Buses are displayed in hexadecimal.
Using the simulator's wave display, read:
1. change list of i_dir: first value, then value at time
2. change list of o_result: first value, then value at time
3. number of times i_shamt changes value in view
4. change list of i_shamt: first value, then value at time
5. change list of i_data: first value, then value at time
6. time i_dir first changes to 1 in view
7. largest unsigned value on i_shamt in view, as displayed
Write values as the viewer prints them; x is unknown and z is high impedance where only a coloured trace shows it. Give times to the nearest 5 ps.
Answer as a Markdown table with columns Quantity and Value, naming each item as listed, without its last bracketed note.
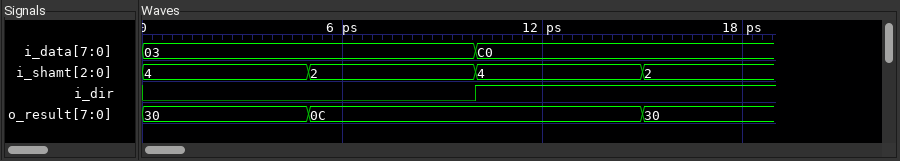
| Quantity | Value |
|---|---|
| change list of i_dir: first value, then value at time | 0, 1 at 10 ps |
| change list of o_result: first value, then value at time | 30, 0C at 5 ps, 30 at 15 ps |
| number of times i_shamt changes value in view | 3 |
| change list of i_shamt: first value, then value at time | 4, 2 at 5 ps, 4 at 10 ps, 2 at 15 ps |
| change list of i_data: first value, then value at time | 03, C0 at 10 ps |
| time i_dir first changes to 1 in view | 10 ps |
| largest unsigned value on i_shamt in view, as displayed | 4 |
